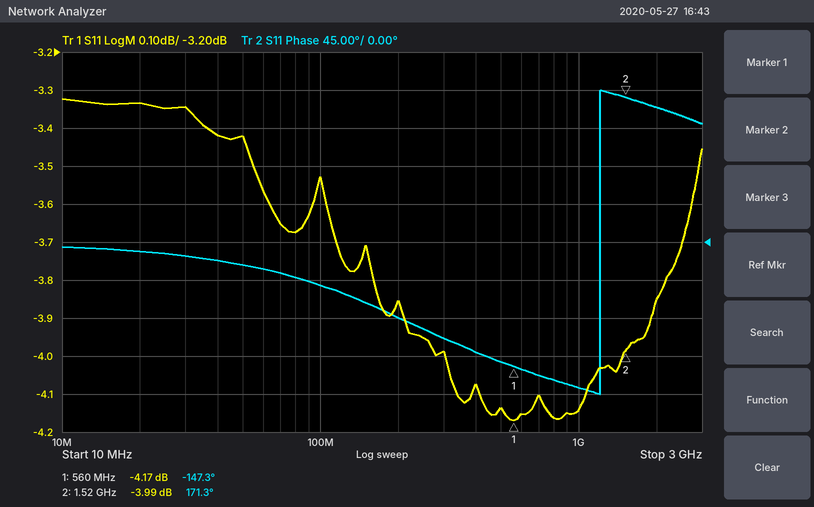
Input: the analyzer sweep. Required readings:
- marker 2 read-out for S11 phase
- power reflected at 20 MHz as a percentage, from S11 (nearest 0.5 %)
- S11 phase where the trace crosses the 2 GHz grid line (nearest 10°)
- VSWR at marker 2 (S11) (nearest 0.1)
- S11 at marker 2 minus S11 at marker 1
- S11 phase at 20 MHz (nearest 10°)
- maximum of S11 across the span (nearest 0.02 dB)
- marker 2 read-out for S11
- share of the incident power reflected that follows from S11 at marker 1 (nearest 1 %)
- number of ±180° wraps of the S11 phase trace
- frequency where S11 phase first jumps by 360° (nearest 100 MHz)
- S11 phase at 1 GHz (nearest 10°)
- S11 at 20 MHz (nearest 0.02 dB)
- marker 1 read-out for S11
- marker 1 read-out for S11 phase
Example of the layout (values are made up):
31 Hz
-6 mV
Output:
171.3°
46.5 %
160°
4.4
0.18 dB
-10°
-3.32 dB
-3.99 dB
38 %
1
1.2 GHz
-170°
-3.34 dB
-4.17 dB
-147.3°
